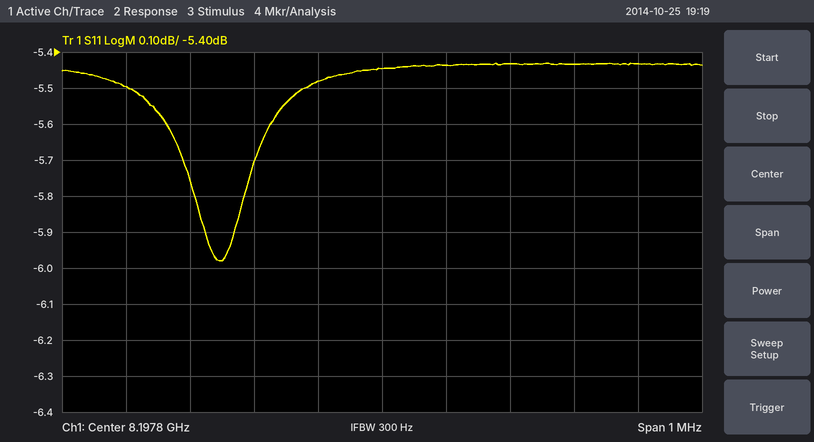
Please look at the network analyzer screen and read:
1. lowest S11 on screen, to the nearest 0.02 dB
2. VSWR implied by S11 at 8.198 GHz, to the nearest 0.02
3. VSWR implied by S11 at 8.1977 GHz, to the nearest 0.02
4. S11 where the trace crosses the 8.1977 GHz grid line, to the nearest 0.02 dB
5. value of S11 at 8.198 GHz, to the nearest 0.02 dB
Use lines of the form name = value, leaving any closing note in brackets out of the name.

lowest S11 on screen, to the nearest 0.02 dB = -5.98 dB
VSWR implied by S11 at 8.198 GHz, to the nearest 0.02 = 3.30
VSWR implied by S11 at 8.1977 GHz, to the nearest 0.02 = 3.28
S11 where the trace crosses the 8.1977 GHz grid line, to the nearest 0.02 dB = -5.48 dB
value of S11 at 8.198 GHz, to the nearest 0.02 dB = -5.44 dB
